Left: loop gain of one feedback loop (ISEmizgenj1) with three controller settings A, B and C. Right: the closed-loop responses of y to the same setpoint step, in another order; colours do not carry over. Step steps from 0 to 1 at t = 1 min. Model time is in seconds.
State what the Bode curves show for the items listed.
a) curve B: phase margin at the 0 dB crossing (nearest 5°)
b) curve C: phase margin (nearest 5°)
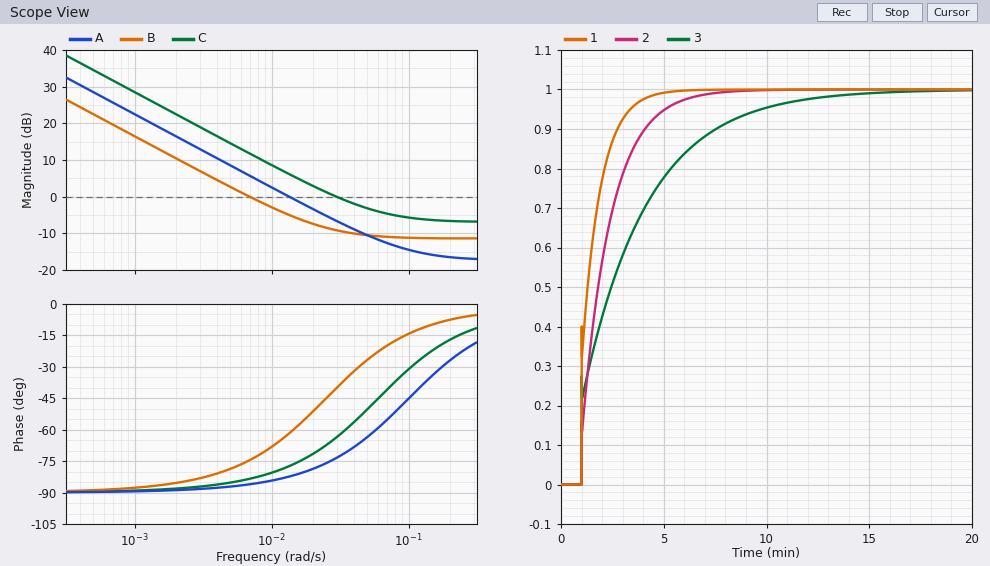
105°
115°
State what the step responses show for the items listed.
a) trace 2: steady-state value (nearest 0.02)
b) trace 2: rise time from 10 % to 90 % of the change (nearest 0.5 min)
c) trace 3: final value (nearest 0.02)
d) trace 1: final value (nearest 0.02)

1.00
3.0 min
1.00
1.00
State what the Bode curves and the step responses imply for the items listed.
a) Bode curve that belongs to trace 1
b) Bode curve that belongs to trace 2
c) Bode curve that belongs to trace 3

C
A
B
